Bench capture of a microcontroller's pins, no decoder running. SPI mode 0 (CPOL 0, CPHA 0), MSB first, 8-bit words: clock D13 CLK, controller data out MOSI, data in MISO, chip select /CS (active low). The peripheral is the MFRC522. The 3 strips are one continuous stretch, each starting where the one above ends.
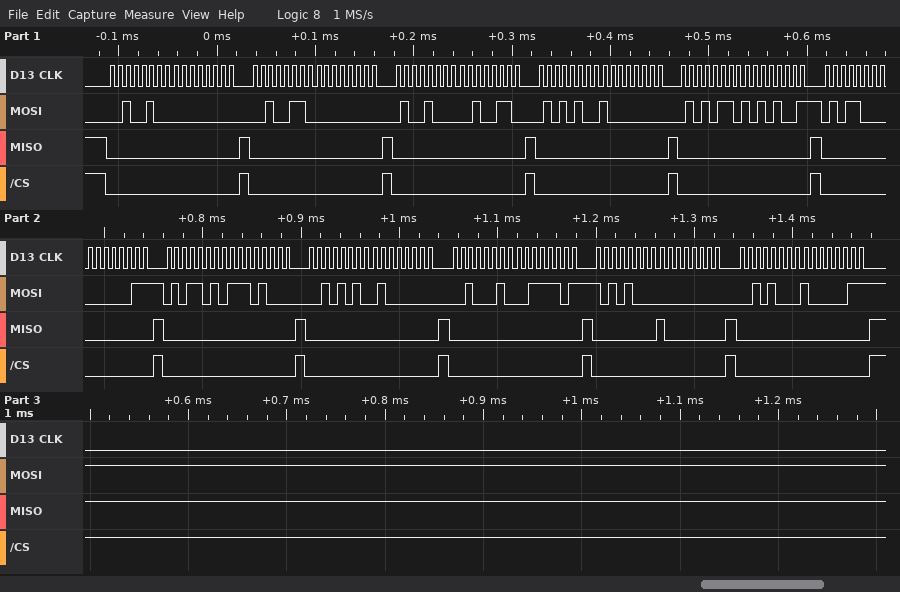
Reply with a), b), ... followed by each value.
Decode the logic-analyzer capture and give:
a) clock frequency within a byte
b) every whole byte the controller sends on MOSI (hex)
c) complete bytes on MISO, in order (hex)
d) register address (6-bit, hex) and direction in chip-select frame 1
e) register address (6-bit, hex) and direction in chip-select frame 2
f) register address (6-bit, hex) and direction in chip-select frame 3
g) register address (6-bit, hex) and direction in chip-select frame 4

a) 125 kHz
b) 0x24 0x00 0x26 0x00 0x48 0x26 0x54 0x80 0x56 0xA9 0x58 0x03 0x5A 0xE8 0x2A 0x40 0x22 0x3D 0xA8 0x00 0x28 0x83
c) 0x00 0x00 0x00 0x00 0x00 0x00 0x00 0x00 0x00 0x00 0x00 0x00 0x00 0x00 0x00 0x00 0x00 0x00 0x00 0x80 0x00 0x00
d) 0x12 write
e) 0x13 write
f) 0x24 write
g) 0x2A write
